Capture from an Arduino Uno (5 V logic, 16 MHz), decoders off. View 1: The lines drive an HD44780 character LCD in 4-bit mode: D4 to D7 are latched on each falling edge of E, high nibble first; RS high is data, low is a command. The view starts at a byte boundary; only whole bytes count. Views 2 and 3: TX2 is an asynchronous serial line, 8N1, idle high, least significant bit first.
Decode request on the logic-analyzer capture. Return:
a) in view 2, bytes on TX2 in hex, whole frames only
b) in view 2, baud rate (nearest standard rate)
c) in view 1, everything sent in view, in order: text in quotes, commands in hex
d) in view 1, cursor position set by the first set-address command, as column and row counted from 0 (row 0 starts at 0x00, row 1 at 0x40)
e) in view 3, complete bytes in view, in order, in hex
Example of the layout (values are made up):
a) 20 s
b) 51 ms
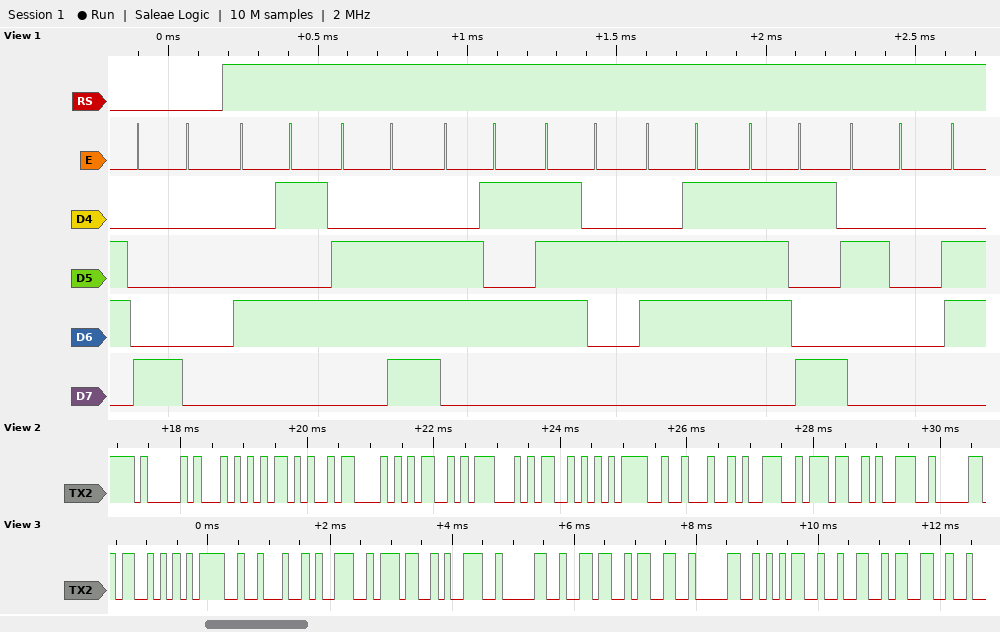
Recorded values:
a) 41 54 2B 43 4D 47 53 3D 22 39 37 39
b) 9600 baud
c) 0x80 "Energy "
d) column 0, row 0
e) 53 3D 22 39 37 39 30 36 33 30 35 32 33
